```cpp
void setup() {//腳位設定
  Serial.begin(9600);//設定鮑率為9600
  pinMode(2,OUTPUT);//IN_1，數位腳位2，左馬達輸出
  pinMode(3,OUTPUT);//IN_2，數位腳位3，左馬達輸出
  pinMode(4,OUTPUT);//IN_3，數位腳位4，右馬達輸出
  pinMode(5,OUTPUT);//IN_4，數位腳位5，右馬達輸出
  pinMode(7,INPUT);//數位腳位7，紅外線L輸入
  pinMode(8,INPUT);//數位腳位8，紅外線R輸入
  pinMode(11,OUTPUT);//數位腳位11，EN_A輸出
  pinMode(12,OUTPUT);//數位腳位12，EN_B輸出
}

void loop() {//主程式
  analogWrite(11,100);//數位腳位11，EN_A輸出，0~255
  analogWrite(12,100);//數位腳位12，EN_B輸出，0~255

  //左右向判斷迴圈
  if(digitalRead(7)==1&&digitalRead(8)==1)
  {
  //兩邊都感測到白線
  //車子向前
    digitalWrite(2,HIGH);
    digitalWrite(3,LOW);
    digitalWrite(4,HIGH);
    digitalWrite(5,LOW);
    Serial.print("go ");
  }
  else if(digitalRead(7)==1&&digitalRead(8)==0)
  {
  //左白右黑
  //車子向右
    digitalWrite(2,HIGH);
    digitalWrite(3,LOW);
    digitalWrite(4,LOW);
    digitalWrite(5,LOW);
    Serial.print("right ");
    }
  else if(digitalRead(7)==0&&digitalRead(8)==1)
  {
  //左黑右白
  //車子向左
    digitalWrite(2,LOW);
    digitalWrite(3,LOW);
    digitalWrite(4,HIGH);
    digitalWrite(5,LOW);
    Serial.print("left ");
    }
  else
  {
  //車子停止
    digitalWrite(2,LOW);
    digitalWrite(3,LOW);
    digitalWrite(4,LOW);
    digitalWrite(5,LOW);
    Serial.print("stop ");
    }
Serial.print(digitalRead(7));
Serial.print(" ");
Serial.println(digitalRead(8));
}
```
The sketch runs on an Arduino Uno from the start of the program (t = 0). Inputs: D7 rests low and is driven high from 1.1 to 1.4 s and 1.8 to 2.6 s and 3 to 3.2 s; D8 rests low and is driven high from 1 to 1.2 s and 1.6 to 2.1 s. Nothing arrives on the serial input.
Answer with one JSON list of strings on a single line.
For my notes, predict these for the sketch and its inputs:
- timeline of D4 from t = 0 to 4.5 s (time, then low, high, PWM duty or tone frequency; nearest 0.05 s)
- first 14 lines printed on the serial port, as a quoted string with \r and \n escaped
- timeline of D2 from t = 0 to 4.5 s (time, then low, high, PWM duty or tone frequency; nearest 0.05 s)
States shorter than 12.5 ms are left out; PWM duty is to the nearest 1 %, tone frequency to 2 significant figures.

["0 s low; 1 s high; 1.2 s low; 1.6 s high; 2.1 s low", "\"stop 0 0\\r\\nstop 0 0\\r\\nstop 0 0\\r\\nstop 0 0\\r\\nstop 0 0\\r\\nstop 0 0\\r\\nstop 0 0\\r\\nstop 0 0\\r\\nstop 0 0\\r\\nstop 0 0\\r\\nstop 0 0\\r\\nstop 0 0\\r\\nstop 0 0\\r\\nstop 0 0\\r\\n\"", "0 s low; 1.1 s high; 1.4 s low; 1.8 s high; 2.6 s low; 3 s high; 3.2 s low"]
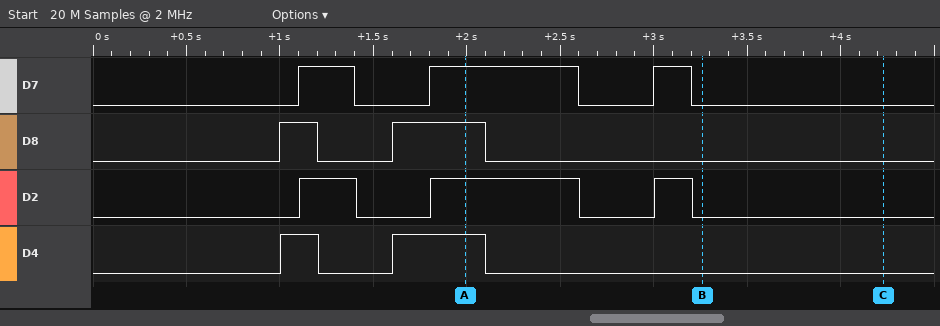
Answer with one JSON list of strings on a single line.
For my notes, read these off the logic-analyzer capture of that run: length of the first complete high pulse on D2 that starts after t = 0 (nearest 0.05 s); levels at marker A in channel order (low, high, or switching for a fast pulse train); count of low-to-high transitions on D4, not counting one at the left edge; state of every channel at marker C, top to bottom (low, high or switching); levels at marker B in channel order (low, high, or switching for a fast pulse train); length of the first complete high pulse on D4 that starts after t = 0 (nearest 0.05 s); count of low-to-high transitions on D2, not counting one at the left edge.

["0.30 s", "D7 high, D8 high, D2 high, D4 high", "2", "D7 low, D8 low, D2 low, D4 low", "D7 low, D8 low, D2 low, D4 low", "0.20 s", "3"]
